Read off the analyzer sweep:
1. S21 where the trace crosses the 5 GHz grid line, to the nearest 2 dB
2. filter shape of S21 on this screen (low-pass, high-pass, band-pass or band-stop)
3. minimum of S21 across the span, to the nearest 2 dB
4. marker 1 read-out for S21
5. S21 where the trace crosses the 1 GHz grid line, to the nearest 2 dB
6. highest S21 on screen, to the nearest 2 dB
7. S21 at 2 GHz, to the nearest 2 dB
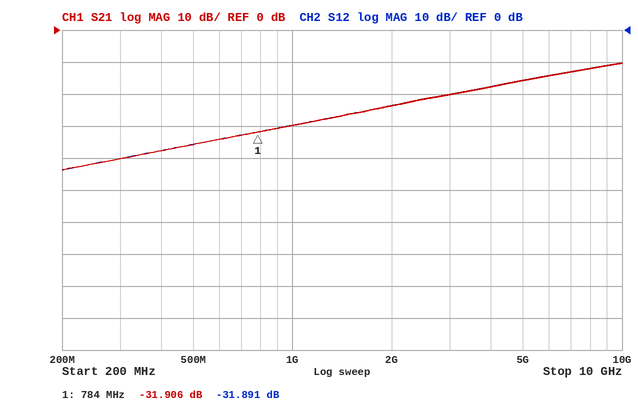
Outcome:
-16 dB
high-pass
-44 dB
-31.906 dB
-30 dB
-10 dB
-24 dB
